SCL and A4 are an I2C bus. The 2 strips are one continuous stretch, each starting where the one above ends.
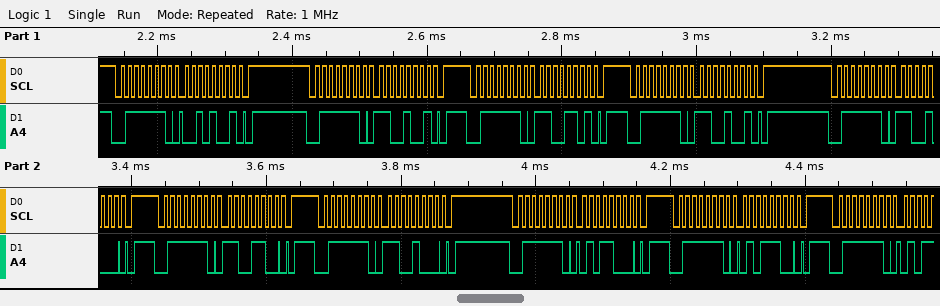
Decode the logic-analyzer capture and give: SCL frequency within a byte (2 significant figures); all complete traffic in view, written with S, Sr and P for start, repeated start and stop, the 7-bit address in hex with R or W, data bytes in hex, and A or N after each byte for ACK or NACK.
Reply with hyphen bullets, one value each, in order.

- 100 kHz
- S 3FW A 29 A P S 3FW A C9 A P S 3FW A CD A P S 3FW A C9 A P S 3FW A C8 A P S 3FW A CC A P S 3FW A C8 A P S 3FW A 58 A P S 3FW A 5C A P S 3FW A
